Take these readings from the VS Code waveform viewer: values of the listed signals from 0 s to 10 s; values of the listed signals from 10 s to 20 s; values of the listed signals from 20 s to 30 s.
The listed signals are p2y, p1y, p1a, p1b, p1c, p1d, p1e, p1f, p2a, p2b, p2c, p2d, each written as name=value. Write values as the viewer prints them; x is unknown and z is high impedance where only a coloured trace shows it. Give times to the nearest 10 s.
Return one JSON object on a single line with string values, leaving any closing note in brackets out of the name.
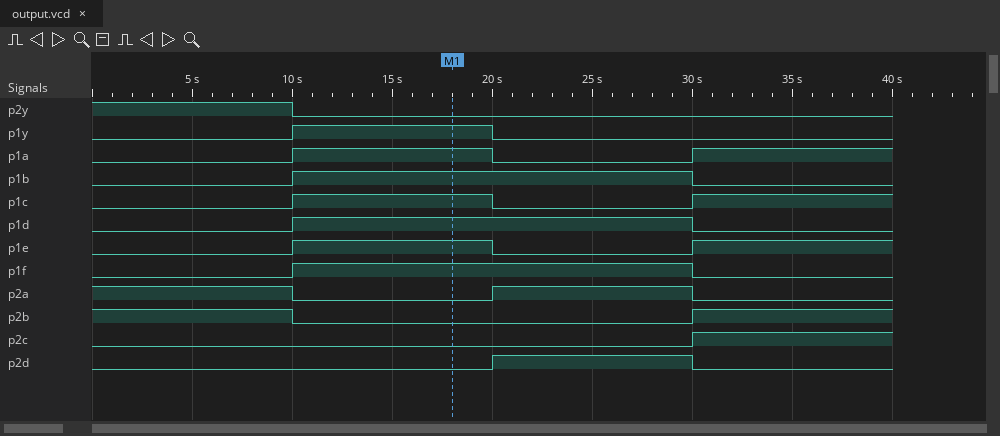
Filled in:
{"values of the listed signals from 0 s to 10 s": "p2y=1, p1y=0, p1a=0, p1b=0, p1c=0, p1d=0, p1e=0, p1f=0, p2a=1, p2b=1, p2c=0, p2d=0", "values of the listed signals from 10 s to 20 s": "p2y=0, p1y=1, p1a=1, p1b=1, p1c=1, p1d=1, p1e=1, p1f=1, p2a=0, p2b=0, p2c=0, p2d=0", "values of the listed signals from 20 s to 30 s": "p2y=0, p1y=0, p1a=0, p1b=1, p1c=0, p1d=1, p1e=0, p1f=1, p2a=1, p2b=0, p2c=0, p2d=1"}
